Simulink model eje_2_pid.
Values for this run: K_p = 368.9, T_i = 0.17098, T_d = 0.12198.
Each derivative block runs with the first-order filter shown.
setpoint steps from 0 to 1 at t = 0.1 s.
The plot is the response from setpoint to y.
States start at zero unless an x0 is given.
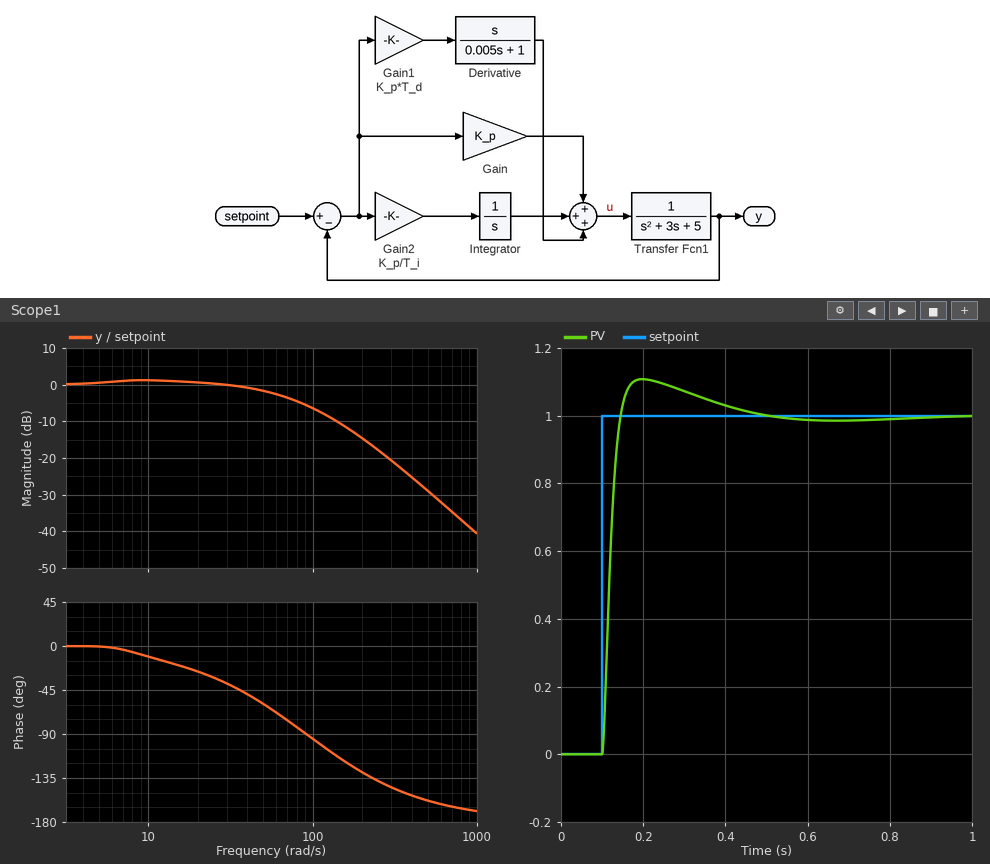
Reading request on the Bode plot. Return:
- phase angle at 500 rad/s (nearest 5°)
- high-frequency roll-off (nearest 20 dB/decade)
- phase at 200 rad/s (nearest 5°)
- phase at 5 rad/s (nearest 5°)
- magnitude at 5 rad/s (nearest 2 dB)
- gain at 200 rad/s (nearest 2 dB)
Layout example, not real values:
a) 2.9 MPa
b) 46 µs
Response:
a) -160°
b) -40 dB/decade
c) -130°
d) 0°
e) 0 dB
f) -14 dB
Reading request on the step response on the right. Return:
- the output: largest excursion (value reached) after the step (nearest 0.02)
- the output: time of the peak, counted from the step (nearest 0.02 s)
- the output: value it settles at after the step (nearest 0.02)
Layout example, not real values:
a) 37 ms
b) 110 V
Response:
a) 1.10
b) 0.10 s
c) 1.00
